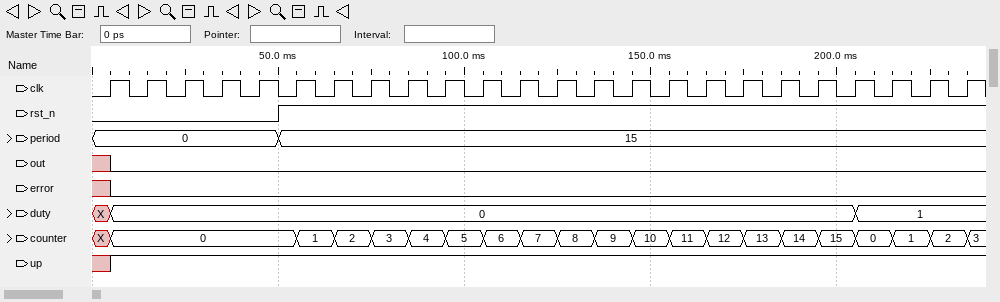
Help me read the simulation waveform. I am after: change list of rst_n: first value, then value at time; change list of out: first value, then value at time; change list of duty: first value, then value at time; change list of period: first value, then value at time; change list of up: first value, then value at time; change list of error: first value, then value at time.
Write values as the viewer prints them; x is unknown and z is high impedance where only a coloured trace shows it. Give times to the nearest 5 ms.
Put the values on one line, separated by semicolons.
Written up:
0, 1 at 50 ms; x, 0 at 5 ms; X, 0 at 5 ms, 1 at 205 ms; 0, 15 at 50 ms; x, 1 at 5 ms; x, 0 at 5 ms
